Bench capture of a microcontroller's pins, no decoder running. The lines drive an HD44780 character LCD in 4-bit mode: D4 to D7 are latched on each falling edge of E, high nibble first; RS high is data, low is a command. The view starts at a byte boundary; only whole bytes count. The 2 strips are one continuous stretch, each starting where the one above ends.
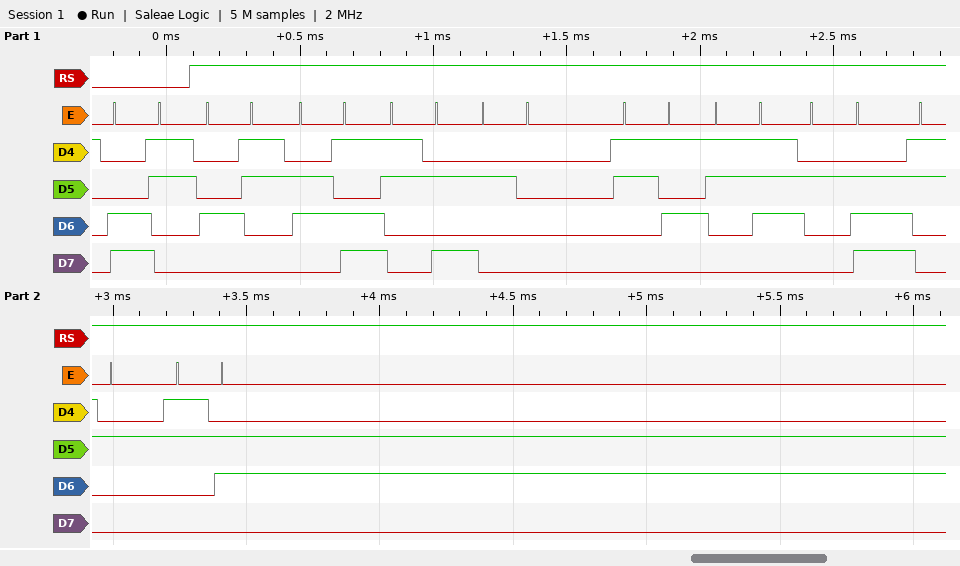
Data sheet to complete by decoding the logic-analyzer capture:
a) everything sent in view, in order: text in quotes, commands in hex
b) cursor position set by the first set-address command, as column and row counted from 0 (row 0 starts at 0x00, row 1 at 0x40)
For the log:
0xC3 "Cm: 57.26"
column 3, row 1
